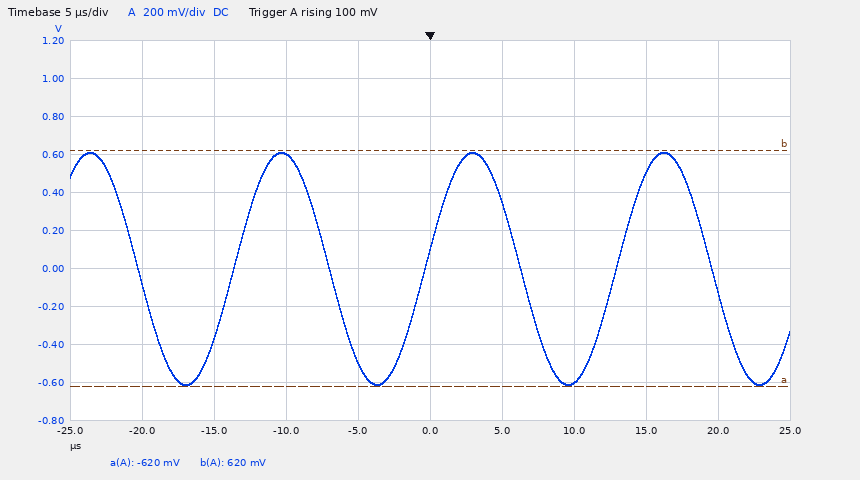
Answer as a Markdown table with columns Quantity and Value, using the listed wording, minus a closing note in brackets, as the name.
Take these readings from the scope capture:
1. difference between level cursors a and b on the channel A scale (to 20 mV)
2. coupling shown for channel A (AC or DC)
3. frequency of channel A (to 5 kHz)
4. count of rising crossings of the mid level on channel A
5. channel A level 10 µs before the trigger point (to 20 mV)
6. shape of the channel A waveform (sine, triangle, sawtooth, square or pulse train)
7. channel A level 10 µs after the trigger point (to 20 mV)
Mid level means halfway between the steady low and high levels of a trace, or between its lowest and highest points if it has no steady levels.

| Quantity | Value |
|---|---|
| difference between level cursors a and b on the channel A scale | 1.24 V |
| coupling shown for channel A | DC |
| frequency of channel A | 75 kHz |
| count of rising crossings of the mid level on channel A | 3 |
| channel A level 10 µs before the trigger point | 600 mV |
| shape of the channel A waveform | sine |
| channel A level 10 µs after the trigger point | -600 mV |
